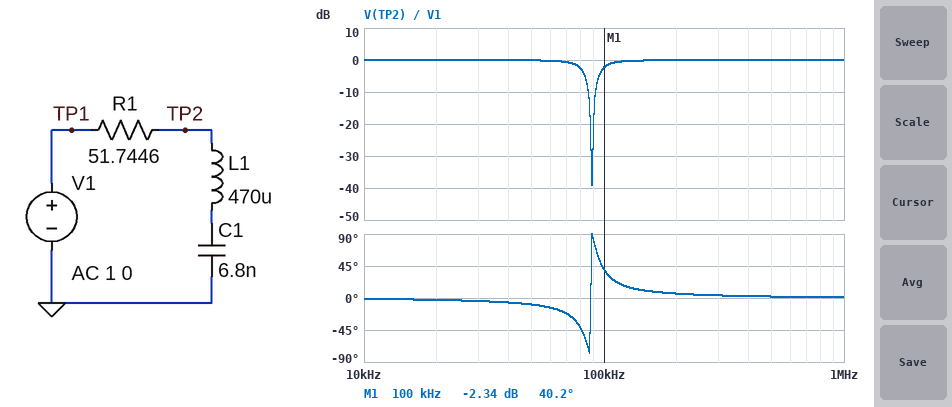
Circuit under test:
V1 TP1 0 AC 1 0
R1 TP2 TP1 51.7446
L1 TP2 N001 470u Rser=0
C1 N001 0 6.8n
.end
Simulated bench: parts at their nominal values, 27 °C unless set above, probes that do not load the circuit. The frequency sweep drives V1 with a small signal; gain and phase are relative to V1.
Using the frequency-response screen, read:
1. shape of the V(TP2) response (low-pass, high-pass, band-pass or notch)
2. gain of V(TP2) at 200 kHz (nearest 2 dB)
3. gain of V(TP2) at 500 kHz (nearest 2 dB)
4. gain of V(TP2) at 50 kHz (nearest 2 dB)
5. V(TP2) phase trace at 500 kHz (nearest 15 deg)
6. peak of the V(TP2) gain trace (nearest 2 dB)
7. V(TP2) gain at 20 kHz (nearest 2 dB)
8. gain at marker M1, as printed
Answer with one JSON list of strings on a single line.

["notch", "0 dB", "0 dB", "0 dB", "0 deg", "0 dB", "0 dB", "-2.34 dB"]
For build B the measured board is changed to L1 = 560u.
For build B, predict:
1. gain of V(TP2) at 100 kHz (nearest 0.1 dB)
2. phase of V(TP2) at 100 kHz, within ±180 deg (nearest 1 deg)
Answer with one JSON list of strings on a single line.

["-0.8 dB", "24 deg"]
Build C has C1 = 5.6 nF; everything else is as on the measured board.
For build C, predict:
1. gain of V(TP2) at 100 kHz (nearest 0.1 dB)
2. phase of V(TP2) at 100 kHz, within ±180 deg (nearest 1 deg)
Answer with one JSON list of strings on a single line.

["-13.6 dB", "78 deg"]
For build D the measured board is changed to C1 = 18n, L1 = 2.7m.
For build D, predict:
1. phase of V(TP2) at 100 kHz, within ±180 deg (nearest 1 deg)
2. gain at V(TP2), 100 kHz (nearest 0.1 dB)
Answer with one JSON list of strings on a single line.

["2 deg", "0 dB"]
